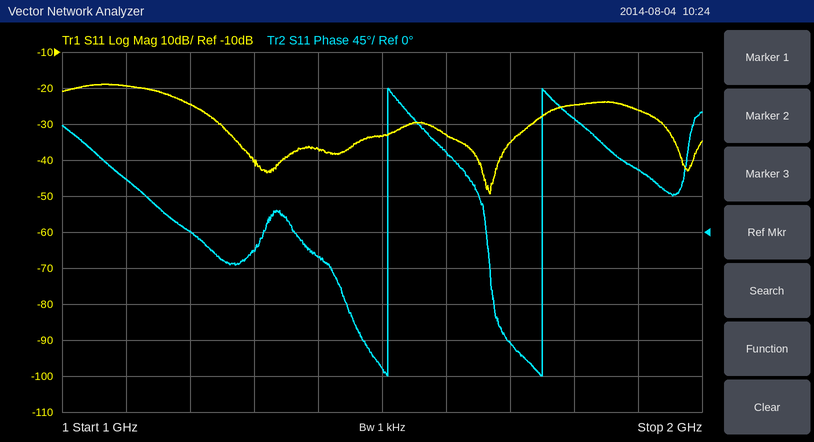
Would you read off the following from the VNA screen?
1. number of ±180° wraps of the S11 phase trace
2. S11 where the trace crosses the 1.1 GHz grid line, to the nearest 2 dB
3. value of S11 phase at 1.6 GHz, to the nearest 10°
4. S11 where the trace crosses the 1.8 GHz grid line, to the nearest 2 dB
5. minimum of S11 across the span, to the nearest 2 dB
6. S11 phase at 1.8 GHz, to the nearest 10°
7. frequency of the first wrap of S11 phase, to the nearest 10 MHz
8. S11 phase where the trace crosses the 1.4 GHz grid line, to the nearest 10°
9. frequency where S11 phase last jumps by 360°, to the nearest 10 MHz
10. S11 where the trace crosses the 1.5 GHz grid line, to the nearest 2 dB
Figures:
2
-20 dB
100°
-24 dB
-50 dB
140°
1.51 GHz
-30°
1.75 GHz
-34 dB
